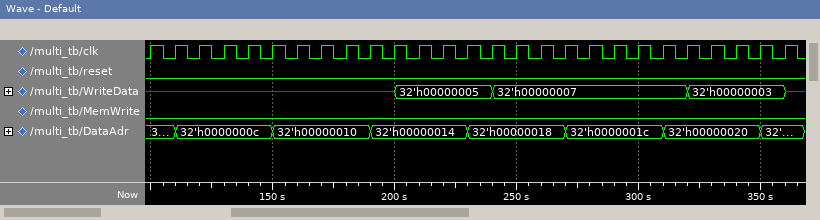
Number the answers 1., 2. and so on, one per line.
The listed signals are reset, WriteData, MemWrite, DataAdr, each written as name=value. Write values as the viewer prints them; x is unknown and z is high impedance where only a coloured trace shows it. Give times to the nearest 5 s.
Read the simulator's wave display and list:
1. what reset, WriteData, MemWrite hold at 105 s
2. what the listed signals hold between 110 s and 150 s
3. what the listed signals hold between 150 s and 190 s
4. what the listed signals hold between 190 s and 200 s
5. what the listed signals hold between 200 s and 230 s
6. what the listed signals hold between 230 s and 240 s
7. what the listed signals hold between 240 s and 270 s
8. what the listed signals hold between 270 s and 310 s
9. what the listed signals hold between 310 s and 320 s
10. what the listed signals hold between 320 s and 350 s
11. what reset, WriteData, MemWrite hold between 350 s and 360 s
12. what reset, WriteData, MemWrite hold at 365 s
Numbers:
1. reset=0, WriteData=x, MemWrite=0
2. reset=0, WriteData=x, MemWrite=0, DataAdr=32'h0000000c
3. reset=0, WriteData=x, MemWrite=0, DataAdr=32'h00000010
4. reset=0, WriteData=x, MemWrite=0, DataAdr=32'h00000014
5. reset=0, WriteData=32'h00000005, MemWrite=0, DataAdr=32'h00000014
6. reset=0, WriteData=32'h00000005, MemWrite=0, DataAdr=32'h00000018
7. reset=0, WriteData=32'h00000007, MemWrite=0, DataAdr=32'h00000018
8. reset=0, WriteData=32'h00000007, MemWrite=0, DataAdr=32'h0000001c
9. reset=0, WriteData=32'h00000007, MemWrite=0, DataAdr=32'h00000020
10. reset=0, WriteData=32'h00000003, MemWrite=0, DataAdr=32'h00000020
11. reset=0, WriteData=32'h00000003, MemWrite=0
12. reset=0, WriteData=x, MemWrite=0
